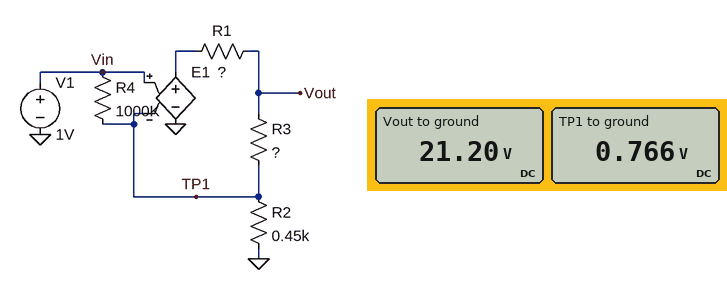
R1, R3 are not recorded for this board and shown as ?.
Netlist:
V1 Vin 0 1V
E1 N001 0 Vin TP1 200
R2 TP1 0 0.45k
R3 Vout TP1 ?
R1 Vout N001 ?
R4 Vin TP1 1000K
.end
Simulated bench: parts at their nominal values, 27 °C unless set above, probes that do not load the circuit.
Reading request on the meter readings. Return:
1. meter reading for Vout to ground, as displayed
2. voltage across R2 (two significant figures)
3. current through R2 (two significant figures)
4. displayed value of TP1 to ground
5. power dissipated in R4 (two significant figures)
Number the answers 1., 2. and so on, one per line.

1. 21.20 V
2. 770 mV
3. 1.7 mA
4. 0.766 V
5. 55 nW
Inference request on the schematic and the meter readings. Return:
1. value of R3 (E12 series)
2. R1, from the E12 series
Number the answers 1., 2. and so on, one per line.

1. 12 kΩ
2. 15 kΩ
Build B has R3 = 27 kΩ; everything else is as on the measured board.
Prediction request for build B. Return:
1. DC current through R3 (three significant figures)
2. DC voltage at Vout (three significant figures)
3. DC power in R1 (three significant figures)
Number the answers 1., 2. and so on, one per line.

1. 1.51 mA
2. 41.4 V
3. 34.2 mW
